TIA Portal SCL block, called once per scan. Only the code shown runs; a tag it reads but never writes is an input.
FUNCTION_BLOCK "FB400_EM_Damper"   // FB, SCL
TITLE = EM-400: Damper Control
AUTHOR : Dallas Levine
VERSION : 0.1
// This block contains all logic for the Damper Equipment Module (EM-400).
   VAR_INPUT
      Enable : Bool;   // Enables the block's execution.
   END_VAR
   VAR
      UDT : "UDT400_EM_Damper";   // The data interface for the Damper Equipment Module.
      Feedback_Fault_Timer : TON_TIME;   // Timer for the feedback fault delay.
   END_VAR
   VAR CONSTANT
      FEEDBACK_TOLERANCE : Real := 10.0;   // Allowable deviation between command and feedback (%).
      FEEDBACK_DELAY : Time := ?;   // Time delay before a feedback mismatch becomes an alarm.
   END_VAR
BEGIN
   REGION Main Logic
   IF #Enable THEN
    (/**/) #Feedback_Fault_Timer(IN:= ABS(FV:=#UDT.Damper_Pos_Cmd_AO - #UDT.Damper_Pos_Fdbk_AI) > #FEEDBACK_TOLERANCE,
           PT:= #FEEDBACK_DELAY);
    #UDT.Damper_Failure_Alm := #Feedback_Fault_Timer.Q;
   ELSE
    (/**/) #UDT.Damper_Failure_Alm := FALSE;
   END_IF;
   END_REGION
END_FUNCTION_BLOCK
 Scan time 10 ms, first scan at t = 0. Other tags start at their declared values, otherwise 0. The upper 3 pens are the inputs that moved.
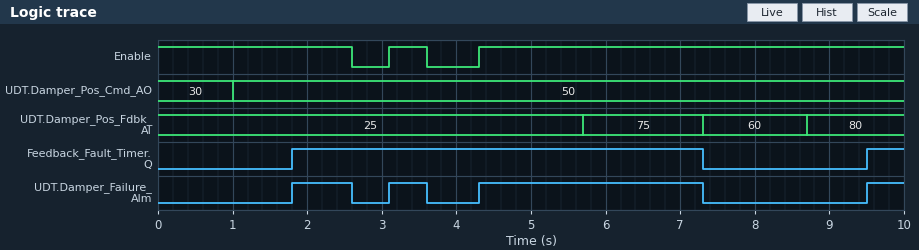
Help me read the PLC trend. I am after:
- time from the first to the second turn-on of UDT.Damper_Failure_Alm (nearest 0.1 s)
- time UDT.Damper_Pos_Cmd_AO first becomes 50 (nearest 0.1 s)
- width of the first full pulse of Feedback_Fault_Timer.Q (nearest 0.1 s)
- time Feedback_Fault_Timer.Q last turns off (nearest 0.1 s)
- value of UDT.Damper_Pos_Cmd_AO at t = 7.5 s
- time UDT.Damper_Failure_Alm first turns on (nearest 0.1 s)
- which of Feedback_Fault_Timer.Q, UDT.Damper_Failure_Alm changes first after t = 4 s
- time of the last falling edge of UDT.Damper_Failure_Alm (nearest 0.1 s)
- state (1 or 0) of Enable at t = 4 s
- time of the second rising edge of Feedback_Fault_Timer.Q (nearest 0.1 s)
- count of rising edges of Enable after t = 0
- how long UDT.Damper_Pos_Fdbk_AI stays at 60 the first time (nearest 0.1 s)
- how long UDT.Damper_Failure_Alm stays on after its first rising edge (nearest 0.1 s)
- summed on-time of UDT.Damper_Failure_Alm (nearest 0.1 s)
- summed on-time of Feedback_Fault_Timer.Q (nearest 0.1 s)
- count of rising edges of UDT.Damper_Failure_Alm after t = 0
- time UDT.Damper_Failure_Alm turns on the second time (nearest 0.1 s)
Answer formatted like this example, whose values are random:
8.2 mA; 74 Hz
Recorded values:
1.3 s; 1.0 s; 5.5 s; 7.3 s; 50; 1.8 s; UDT.Damper_Failure_Alm; 7.3 s; 0; 9.5 s; 2; 1.4 s; 0.8 s; 4.8 s; 6.0 s; 4; 3.1 s
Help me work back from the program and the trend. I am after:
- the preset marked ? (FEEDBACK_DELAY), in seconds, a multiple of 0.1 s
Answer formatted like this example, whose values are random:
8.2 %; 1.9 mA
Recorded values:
0.8 s
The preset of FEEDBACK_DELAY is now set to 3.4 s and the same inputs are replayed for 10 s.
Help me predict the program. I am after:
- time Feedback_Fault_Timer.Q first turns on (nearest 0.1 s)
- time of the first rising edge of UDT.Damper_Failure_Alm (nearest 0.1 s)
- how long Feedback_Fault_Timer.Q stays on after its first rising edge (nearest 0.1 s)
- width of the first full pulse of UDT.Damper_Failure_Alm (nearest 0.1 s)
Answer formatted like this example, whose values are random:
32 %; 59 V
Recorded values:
4.4 s; 4.4 s; 2.9 s; 2.9 s
